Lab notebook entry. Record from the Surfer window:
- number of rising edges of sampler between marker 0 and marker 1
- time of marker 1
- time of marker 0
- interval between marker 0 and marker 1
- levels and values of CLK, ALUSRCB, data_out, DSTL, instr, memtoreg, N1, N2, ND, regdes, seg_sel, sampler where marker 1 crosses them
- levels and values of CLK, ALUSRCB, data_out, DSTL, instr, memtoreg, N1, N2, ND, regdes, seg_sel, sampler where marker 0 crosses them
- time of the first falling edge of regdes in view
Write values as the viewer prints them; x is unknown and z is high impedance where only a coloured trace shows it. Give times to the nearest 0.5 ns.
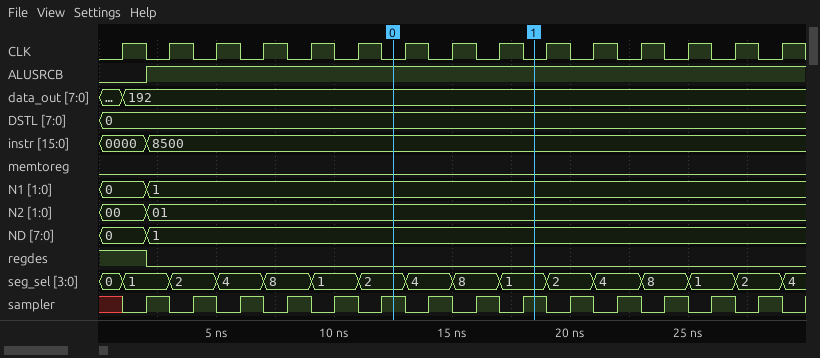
3
18.5 ns
12.5 ns
6 ns
CLK=0, ALUSRCB=1, data_out=192, DSTL=0, instr=8500, memtoreg=0, N1=1, N2=01, ND=1, regdes=0, seg_sel=1, sampler=1
CLK=0, ALUSRCB=1, data_out=192, DSTL=0, instr=8500, memtoreg=0, N1=1, N2=01, ND=1, regdes=0, seg_sel=2, sampler=1
2 ns
